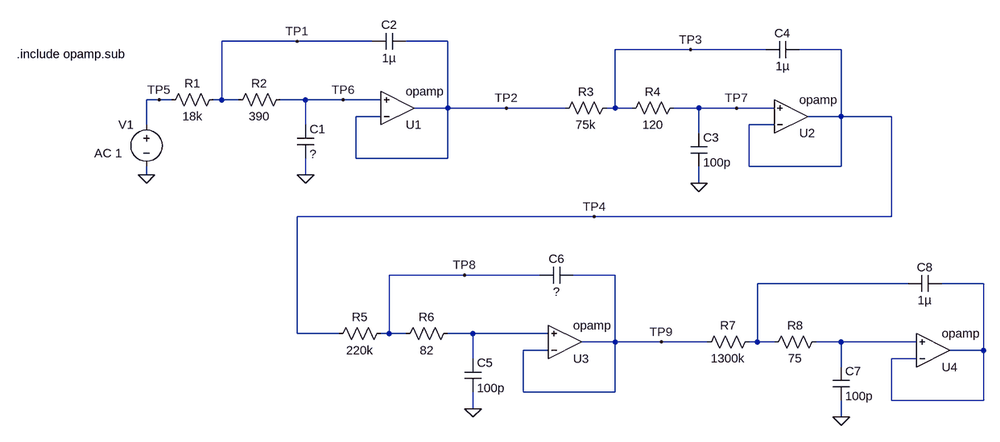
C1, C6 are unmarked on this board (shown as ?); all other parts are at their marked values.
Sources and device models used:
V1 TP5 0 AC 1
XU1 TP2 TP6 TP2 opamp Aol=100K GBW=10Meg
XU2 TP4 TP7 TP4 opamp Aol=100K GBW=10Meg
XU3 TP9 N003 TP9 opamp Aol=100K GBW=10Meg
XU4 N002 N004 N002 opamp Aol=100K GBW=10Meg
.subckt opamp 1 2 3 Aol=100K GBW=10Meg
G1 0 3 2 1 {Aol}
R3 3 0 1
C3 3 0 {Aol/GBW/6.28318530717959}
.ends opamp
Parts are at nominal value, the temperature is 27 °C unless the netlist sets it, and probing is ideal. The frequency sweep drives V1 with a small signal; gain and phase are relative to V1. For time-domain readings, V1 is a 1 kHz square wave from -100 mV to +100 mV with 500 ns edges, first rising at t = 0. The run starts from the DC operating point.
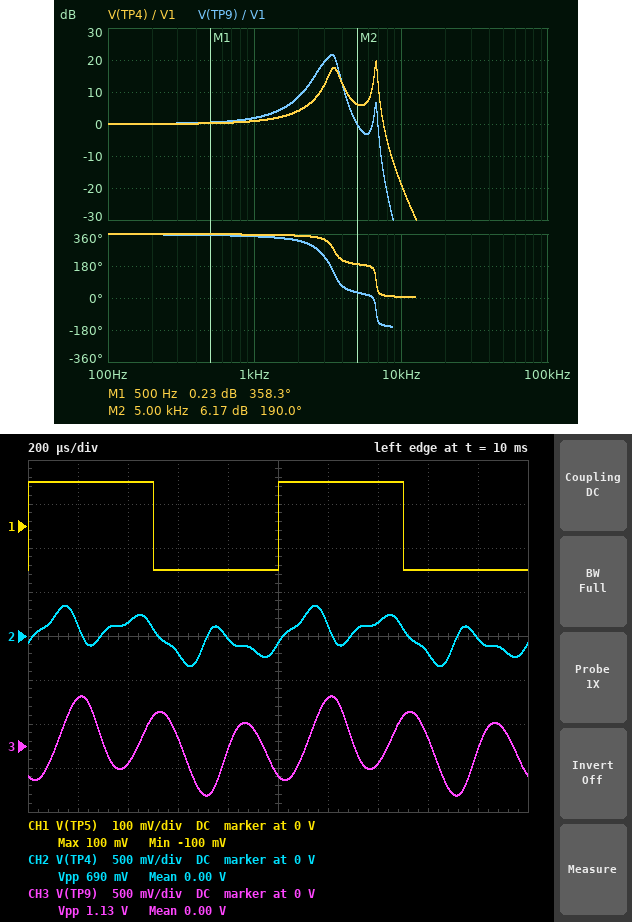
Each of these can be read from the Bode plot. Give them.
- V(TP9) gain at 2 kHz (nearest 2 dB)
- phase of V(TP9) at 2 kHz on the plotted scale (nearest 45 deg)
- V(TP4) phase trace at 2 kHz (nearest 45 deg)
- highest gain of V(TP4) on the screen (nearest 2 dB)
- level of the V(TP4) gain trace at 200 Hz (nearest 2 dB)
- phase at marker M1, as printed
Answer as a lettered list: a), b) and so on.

a) 8 dB
b) 315 deg
c) 360 deg
d) 20 dB
e) 0 dB
f) 358.3 deg
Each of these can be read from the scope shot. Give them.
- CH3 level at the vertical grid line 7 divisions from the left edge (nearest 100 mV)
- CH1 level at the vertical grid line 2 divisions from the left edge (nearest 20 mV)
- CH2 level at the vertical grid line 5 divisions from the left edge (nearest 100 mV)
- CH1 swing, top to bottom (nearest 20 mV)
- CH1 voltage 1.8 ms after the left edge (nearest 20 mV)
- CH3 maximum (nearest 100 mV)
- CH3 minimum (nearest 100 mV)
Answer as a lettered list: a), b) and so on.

a) -200 mV
b) 100 mV
c) -100 mV
d) 200 mV
e) -100 mV
f) 600 mV
g) -600 mV
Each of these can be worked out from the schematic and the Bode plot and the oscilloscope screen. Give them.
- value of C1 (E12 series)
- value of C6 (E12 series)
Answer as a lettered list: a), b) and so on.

a) 39 pF
b) 560 nF
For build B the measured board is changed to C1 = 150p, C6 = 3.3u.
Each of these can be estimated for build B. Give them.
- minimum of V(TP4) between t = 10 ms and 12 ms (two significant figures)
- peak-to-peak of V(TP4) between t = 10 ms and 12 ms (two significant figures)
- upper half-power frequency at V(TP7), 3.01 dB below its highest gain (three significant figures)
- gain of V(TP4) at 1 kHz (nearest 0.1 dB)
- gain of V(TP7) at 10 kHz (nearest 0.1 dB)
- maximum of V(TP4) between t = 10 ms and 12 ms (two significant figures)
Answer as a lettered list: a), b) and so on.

a) -400 mV
b) 790 mV
c) 4.46 kHz
d) 1.2 dB
e) -29.9 dB
f) 400 mV
